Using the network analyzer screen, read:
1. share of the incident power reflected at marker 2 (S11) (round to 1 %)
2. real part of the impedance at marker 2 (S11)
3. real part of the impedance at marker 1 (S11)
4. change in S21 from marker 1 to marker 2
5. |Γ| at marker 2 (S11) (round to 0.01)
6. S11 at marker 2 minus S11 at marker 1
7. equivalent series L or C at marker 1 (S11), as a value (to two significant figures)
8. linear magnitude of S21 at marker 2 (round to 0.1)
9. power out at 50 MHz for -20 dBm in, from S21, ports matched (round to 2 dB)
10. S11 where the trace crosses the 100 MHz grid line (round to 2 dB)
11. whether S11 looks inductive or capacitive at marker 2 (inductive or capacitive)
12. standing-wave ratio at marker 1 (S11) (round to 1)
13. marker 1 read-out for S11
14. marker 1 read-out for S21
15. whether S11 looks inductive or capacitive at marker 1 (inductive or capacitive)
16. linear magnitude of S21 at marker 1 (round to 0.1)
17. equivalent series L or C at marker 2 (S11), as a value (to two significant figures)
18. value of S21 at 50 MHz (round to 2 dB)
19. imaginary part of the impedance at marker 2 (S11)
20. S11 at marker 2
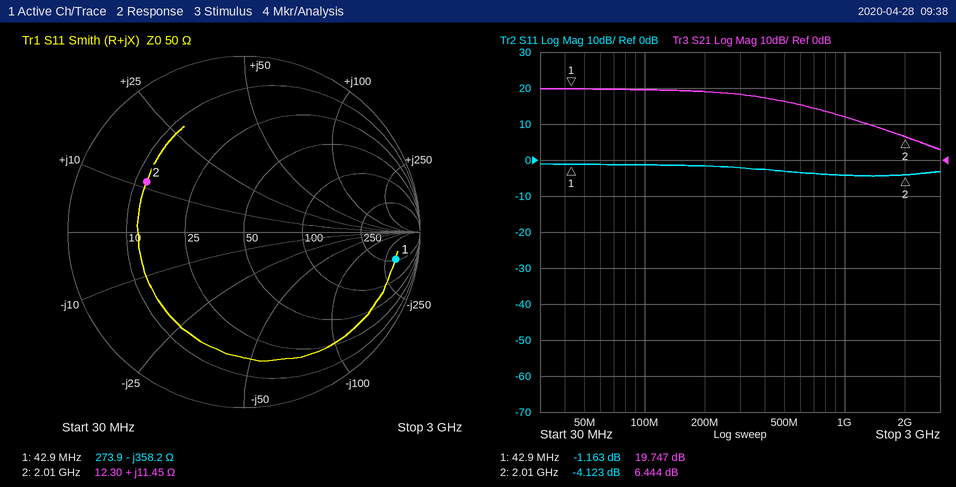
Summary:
39 %
12.30 Ω
273.9 Ω
-13.303 dB
0.62
-2.960 dB
10 pF
2.1
0 dBm
-2 dB
inductive
15
-1.163 dB
19.747 dB
capacitive
9.7
910 pH
20 dB
+11.45 Ω
-4.123 dB
